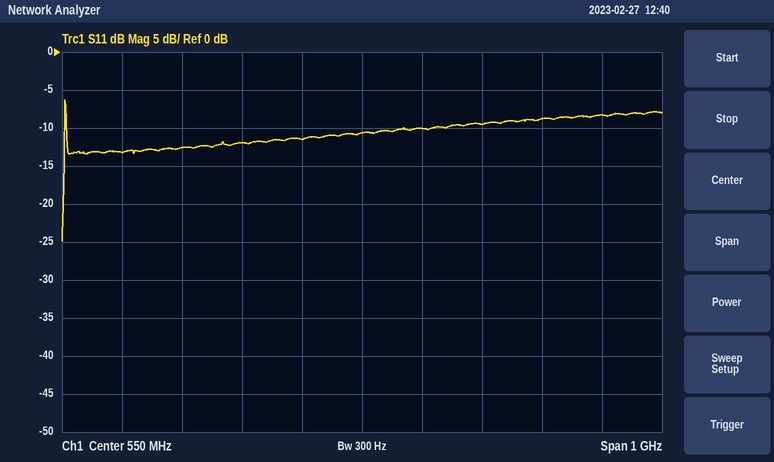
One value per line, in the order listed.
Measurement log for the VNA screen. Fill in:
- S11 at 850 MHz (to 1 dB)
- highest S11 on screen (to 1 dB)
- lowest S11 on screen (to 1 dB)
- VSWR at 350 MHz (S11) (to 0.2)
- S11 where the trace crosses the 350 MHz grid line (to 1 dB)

-9 dB
-6 dB
-25 dB
1.6
-12 dB
